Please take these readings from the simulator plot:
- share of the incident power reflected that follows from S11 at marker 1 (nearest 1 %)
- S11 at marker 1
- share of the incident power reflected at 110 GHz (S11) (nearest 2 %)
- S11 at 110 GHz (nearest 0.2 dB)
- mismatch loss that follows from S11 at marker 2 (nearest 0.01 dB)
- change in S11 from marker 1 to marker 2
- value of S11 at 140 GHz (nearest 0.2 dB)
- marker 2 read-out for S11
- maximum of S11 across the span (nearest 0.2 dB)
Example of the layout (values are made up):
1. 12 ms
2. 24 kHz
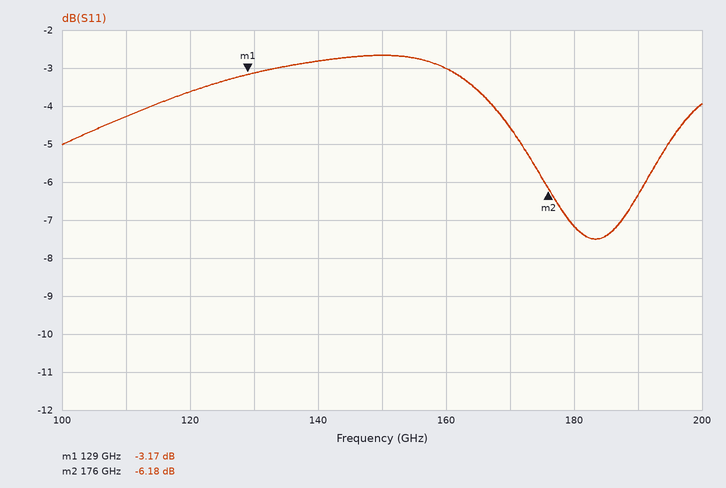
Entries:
1. 48 %
2. -3.17 dB
3. 38 %
4. -4.2 dB
5. 1.20 dB
6. -3.01 dB
7. -2.8 dB
8. -6.18 dB
9. -2.6 dB
